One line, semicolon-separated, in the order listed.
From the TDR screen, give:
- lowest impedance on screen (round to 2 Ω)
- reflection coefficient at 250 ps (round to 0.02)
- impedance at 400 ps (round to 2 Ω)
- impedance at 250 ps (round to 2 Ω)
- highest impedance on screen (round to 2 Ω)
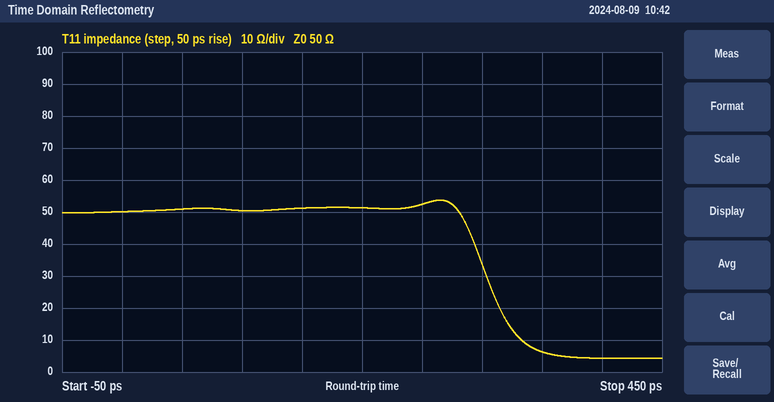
4 Ω; +0.02; 4 Ω; 52 Ω; 54 Ω
